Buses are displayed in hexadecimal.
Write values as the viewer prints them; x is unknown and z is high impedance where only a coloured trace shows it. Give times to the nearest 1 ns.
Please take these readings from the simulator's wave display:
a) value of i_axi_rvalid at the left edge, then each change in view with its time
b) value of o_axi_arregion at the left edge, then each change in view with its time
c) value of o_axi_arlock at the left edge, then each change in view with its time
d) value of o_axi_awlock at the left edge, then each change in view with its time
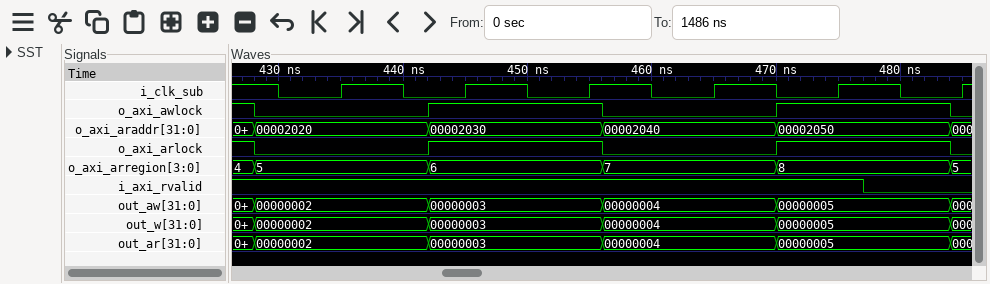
1, 0 at 477 ns
4, 5 at 428 ns, 6 at 442 ns, 7 at 456 ns, 8 at 470 ns, 5 at 484 ns
1, 0 at 428 ns, 1 at 442 ns, 0 at 456 ns, 1 at 470 ns, 0 at 484 ns
1, 0 at 428 ns, 1 at 442 ns, 0 at 456 ns, 1 at 470 ns, 0 at 484 ns
